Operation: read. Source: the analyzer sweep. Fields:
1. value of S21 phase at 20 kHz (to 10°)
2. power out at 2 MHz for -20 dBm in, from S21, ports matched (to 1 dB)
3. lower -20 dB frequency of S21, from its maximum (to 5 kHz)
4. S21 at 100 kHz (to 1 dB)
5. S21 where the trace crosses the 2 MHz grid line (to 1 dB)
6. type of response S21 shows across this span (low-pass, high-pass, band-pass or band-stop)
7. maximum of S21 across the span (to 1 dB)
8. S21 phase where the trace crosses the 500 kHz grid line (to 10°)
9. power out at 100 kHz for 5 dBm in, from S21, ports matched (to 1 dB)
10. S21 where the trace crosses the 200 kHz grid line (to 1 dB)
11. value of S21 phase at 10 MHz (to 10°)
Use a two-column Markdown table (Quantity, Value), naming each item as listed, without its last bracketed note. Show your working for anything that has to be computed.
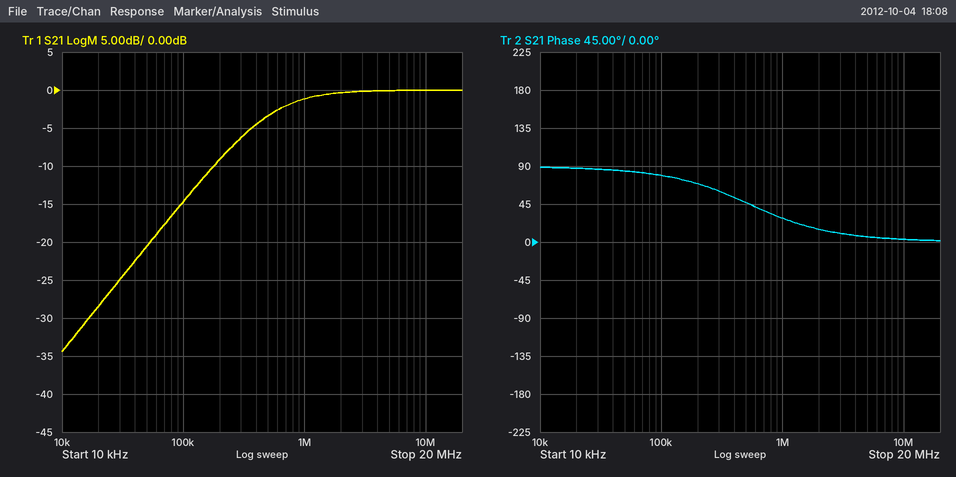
| Quantity | Value |
|---|---|
| value of S21 phase at 20 kHz | 90° |
| power out at 2 MHz for -20 dBm in, from S21, ports matched | -20 dBm + (0 dB) = -20 dBm |
| lower -20 dB frequency of S21, from its maximum | 55 kHz |
| S21 at 100 kHz | -15 dB |
| S21 where the trace crosses the 2 MHz grid line | 0 dB |
| type of response S21 shows across this span | high-pass |
| maximum of S21 across the span | 0 dB |
| S21 phase where the trace crosses the 500 kHz grid line | 50° |
| power out at 100 kHz for 5 dBm in, from S21, ports matched | 5 dBm + (-15 dB) = -10 dBm |
| S21 where the trace crosses the 200 kHz grid line | -9 dB |
| value of S21 phase at 10 MHz | 0° |
